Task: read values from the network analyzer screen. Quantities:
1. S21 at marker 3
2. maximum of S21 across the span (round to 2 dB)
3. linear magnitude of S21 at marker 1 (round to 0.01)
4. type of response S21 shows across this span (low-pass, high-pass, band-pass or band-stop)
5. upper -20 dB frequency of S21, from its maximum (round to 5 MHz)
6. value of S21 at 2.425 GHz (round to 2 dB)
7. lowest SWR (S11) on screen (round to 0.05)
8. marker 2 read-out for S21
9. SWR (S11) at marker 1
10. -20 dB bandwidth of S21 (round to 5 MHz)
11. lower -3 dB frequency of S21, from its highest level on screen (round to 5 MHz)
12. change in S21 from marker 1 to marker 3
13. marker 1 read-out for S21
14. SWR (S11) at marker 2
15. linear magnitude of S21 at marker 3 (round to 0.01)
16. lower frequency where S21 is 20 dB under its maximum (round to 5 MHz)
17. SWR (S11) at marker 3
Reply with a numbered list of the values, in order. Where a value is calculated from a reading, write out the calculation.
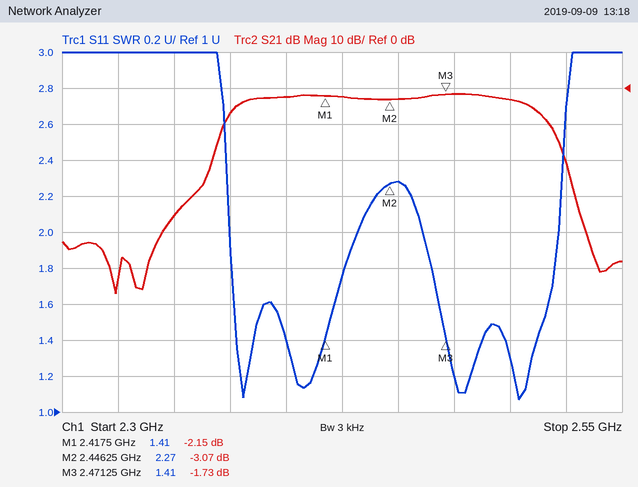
1. -1.73 dB
2. -2 dB
3. 10^(-2.15/20) ≈ 0.78
4. band-pass
5. 2.525 GHz
6. -2 dB
7. 1.05
8. -3.07 dB
9. 1.41
10. 2.525 GHz − 2.365 GHz = 160 MHz
11. 2.380 GHz
12. -1.73 − (-2.15) = 0.42 dB
13. -2.15 dB
14. 2.27
15. 10^(-1.73/20) ≈ 0.82
16. 2.365 GHz
17. 1.41
